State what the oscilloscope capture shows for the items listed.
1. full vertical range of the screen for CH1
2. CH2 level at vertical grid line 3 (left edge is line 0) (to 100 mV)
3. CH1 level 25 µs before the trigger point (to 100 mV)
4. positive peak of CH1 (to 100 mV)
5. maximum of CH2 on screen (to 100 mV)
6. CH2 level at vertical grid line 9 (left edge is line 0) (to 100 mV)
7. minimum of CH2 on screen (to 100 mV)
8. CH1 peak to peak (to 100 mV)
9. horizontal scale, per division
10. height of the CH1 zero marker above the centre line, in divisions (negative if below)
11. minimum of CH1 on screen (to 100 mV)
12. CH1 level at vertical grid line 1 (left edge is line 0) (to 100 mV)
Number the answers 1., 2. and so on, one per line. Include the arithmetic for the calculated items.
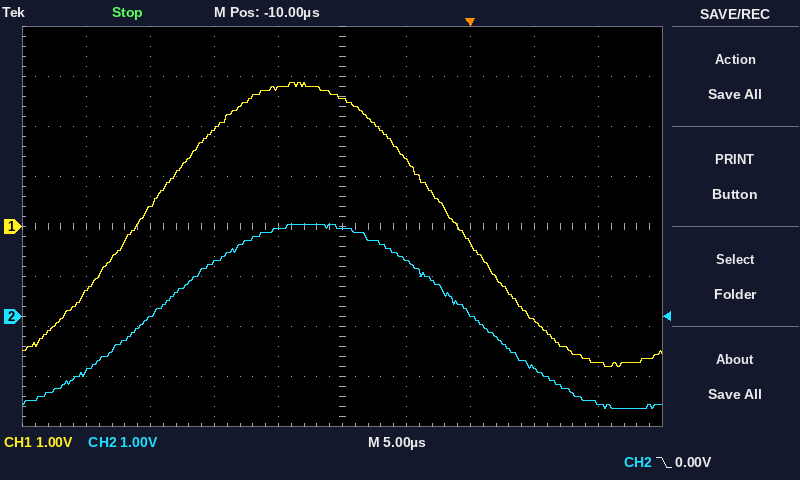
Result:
1. 8 V
2. 1.1 V
3. 400 mV
4. 2.9 V
5. 1.8 V
6. -1.7 V
7. -1.8 V
8. 2.9 V − (-2.8 V) = 5.7 V
9. 5 µs
10. 0.0 div
11. -2.8 V
12. -1.3 V
